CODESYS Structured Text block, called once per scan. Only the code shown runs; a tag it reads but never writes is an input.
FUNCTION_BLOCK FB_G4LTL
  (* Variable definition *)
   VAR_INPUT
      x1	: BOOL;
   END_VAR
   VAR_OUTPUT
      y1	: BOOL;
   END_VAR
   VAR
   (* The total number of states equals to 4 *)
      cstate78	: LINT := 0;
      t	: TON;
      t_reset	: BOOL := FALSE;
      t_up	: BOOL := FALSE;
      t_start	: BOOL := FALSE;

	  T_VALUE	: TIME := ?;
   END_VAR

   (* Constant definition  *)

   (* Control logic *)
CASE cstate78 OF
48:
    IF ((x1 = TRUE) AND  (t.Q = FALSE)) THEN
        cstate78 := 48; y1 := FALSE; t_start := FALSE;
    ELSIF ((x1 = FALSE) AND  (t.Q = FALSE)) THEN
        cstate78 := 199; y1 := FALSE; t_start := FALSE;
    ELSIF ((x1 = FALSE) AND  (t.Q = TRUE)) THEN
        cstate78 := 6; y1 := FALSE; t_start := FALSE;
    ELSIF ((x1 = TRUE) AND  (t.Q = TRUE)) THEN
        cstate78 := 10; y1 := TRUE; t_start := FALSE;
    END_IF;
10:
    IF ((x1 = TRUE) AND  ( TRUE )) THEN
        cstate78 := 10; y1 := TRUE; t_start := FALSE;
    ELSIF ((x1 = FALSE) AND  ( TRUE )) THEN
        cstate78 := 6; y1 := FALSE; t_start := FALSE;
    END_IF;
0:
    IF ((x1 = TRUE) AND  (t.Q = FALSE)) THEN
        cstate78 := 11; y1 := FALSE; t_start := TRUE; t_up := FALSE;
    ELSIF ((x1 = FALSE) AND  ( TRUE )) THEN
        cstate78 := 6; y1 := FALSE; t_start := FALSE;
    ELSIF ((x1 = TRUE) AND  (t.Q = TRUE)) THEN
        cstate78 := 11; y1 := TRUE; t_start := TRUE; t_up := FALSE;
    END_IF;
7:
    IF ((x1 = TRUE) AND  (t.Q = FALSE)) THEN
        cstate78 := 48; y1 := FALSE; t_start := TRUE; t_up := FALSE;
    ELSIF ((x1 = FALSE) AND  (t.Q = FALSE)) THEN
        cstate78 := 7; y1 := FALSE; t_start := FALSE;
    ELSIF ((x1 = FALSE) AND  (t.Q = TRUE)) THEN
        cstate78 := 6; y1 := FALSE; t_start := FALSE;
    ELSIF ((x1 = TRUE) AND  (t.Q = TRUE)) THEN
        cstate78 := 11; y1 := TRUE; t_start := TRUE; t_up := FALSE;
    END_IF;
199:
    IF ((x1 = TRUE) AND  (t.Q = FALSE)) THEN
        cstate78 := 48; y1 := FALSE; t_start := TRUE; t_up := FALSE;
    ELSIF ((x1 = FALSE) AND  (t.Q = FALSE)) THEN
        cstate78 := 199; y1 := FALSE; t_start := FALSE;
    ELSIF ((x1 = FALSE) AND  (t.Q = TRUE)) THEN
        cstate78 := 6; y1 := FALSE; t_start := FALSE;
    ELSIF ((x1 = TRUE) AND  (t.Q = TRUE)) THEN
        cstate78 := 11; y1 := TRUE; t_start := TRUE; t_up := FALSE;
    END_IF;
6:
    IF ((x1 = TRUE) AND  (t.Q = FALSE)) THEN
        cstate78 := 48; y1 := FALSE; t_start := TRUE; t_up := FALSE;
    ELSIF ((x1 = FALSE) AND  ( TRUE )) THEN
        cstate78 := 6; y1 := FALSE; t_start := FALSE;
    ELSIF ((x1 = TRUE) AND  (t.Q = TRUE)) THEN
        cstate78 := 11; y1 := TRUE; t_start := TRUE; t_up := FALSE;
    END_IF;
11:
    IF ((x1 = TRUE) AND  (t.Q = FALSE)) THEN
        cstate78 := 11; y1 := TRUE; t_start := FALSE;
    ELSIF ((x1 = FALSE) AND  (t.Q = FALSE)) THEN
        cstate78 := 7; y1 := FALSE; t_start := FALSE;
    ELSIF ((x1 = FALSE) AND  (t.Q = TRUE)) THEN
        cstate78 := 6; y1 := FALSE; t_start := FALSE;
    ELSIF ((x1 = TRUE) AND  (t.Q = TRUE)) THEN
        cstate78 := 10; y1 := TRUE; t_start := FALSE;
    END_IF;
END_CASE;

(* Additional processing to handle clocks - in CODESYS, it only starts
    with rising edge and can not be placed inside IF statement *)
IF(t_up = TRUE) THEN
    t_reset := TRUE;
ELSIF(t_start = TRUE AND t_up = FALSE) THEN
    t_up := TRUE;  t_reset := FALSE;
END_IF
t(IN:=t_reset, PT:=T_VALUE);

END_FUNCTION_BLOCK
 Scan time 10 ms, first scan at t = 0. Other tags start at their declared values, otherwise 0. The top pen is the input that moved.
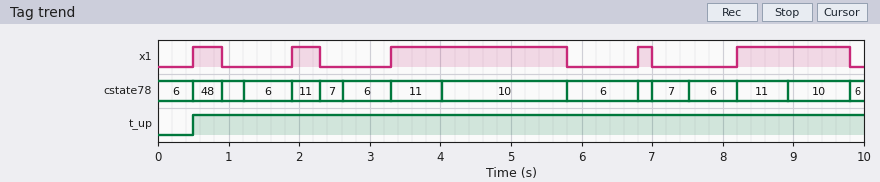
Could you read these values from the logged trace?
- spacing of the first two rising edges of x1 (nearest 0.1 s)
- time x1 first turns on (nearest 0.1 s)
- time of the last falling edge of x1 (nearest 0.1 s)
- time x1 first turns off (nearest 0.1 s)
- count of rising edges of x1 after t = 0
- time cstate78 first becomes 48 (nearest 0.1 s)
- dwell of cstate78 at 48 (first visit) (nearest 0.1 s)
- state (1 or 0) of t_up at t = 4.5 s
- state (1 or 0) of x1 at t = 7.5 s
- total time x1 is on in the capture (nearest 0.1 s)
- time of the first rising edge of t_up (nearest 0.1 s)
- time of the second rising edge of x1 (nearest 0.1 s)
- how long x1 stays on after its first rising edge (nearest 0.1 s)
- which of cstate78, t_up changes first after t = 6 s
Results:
1.4 s
0.5 s
9.8 s
0.9 s
5
0.5 s
0.4 s
1
0
5.1 s
0.5 s
1.9 s
0.4 s
cstate78
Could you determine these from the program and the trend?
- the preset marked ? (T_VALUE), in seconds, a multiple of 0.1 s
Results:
0.7 s
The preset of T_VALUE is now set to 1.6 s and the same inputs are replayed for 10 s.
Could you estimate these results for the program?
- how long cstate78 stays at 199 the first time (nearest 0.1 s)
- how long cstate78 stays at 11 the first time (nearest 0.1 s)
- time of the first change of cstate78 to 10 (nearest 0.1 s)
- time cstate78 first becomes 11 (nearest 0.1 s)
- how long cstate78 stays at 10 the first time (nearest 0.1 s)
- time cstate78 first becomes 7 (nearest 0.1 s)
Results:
1.0 s
0.2 s
4.9 s
6.8 s
0.9 s
7.0 s
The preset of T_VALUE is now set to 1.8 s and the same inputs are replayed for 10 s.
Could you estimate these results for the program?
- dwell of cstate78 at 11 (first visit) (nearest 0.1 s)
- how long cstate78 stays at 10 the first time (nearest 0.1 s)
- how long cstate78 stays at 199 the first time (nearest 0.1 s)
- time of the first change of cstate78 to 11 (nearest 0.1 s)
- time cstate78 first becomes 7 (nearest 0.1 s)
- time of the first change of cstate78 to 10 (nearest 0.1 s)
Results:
0.2 s
0.7 s
1.0 s
6.8 s
7.0 s
5.1 s
